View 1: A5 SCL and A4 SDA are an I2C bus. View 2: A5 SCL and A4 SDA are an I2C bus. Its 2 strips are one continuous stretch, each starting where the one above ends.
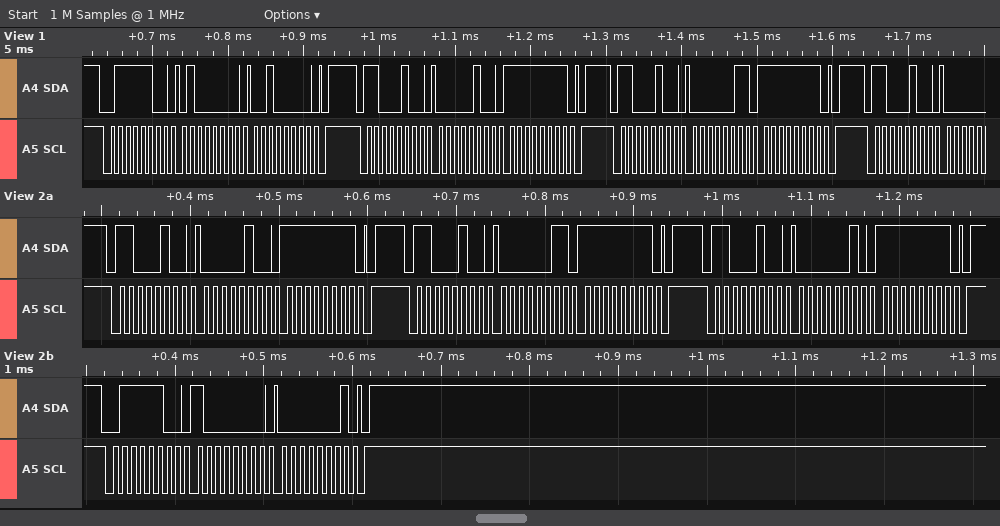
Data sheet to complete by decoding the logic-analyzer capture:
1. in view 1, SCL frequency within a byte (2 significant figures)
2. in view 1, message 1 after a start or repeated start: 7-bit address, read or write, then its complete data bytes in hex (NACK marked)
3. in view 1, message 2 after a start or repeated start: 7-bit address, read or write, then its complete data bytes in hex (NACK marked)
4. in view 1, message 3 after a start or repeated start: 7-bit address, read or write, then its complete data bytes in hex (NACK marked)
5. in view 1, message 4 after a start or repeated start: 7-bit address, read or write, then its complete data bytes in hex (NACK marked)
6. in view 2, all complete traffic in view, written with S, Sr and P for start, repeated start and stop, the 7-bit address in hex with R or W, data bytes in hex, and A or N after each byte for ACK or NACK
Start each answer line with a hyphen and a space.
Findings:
- 100 kHz
- 0x3E write: 40 20
- 0x62 write: 04 FF
- 0x62 write: 03 FF
- 0x62 write
- S 62W A 04 A FF A P S 62W A 03 A FF A P S 62W A 02 A FF A P S 3EW A 80 A 01 A P
